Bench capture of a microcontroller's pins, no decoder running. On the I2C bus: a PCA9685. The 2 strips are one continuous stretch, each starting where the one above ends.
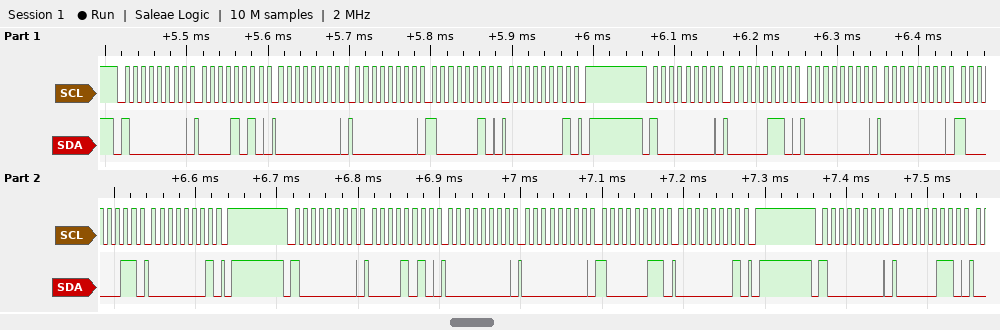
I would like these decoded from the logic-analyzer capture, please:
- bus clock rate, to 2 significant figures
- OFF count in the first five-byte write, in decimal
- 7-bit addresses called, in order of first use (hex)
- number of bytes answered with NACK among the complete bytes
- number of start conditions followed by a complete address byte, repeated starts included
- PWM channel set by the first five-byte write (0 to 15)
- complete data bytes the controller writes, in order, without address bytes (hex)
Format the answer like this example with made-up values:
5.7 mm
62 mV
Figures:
100 kHz
386
0x40
0
4
1
0A 00 00 82 01 06 00 00 83 01 0A 00 00 83 01 06
